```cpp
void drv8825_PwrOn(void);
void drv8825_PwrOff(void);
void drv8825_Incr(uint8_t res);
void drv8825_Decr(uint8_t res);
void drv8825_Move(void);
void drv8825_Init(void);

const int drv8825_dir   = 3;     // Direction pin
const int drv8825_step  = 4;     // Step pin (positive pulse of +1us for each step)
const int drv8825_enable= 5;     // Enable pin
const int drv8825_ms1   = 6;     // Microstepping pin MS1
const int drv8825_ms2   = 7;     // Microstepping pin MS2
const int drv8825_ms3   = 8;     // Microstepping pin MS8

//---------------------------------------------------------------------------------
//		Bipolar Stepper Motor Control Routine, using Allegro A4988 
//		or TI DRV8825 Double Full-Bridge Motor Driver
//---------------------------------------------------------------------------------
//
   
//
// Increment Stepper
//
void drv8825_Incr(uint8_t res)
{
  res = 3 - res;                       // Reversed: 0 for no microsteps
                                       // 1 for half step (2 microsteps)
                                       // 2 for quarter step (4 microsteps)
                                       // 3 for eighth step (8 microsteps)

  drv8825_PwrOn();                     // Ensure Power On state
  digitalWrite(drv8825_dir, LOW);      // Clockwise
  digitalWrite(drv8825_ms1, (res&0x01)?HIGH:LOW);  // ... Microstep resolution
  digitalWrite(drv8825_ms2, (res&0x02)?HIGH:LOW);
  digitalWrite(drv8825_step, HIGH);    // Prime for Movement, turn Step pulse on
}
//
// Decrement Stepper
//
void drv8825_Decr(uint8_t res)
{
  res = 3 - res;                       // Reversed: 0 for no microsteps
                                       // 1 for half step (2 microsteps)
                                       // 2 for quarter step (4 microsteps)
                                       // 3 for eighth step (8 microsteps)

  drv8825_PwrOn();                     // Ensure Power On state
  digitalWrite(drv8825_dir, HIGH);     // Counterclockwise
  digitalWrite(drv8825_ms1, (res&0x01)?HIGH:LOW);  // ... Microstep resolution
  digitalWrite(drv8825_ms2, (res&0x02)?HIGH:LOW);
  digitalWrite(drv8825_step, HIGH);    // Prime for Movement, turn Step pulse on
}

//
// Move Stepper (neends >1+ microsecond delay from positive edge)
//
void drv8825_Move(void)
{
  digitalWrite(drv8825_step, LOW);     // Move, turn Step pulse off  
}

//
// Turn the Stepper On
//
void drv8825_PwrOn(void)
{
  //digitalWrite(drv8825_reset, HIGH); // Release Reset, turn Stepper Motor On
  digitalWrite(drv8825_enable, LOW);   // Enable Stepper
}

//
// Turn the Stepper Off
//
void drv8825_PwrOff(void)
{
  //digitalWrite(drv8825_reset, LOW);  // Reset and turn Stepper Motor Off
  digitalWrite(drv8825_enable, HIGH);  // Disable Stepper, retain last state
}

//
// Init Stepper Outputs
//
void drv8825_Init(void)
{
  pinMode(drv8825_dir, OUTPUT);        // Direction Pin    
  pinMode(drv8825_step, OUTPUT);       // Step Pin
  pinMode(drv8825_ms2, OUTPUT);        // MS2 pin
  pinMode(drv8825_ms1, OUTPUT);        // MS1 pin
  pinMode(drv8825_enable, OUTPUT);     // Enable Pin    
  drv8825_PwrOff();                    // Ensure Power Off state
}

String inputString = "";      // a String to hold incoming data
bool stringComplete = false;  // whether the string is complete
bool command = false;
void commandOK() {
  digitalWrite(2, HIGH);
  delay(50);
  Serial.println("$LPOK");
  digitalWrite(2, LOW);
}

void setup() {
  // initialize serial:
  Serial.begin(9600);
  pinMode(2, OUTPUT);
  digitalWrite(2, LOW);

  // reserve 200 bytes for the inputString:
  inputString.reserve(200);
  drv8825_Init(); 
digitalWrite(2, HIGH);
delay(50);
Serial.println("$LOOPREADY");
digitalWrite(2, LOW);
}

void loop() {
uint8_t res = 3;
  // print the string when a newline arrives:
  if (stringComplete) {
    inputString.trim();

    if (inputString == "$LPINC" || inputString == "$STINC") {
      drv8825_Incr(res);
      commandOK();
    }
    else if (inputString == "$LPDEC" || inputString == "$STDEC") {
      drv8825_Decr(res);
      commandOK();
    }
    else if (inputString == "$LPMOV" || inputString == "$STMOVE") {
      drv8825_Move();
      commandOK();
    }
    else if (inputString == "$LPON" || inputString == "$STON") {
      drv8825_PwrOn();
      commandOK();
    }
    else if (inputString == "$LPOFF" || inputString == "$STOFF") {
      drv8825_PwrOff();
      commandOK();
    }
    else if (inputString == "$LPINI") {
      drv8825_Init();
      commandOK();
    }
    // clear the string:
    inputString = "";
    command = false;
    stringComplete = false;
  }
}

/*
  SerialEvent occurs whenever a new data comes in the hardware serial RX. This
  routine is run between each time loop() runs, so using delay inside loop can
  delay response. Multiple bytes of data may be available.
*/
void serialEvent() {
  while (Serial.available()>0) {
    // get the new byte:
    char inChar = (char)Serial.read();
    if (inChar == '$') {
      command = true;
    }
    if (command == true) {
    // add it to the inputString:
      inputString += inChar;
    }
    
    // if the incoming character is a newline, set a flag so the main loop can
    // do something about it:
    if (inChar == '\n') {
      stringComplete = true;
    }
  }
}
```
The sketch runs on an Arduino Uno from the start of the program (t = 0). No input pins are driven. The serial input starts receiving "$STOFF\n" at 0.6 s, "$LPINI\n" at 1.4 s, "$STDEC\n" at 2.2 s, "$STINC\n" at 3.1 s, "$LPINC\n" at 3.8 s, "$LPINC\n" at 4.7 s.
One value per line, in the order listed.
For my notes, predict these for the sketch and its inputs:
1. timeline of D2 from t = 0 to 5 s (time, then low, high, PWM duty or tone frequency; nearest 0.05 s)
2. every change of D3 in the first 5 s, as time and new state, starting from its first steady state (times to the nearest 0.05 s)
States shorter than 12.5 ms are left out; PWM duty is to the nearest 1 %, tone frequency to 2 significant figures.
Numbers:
0 s high; 0.05 s low; 0.6 s high; 0.65 s low; 1.4 s high; 1.45 s low; 2.2 s high; 2.25 s low; 3.1 s high; 3.15 s low; 3.8 s high; 3.85 s low; 4.7 s high; 4.75 s low
0 s low; 2.2 s high; 3.1 s low
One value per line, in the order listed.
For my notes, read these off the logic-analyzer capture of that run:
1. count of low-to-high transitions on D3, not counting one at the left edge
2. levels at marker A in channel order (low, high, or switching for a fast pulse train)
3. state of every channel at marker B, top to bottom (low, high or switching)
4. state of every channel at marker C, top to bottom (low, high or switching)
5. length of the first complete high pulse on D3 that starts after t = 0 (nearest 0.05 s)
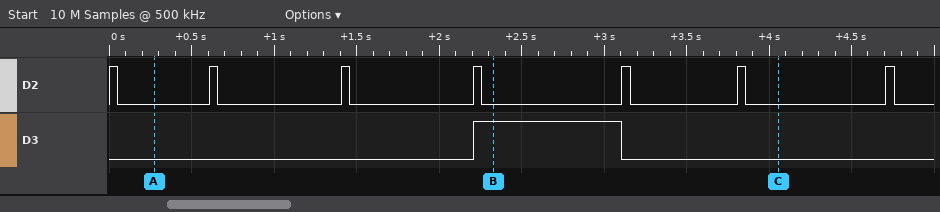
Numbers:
1
D2 low, D3 low
D2 low, D3 high
D2 low, D3 low
0.90 s
